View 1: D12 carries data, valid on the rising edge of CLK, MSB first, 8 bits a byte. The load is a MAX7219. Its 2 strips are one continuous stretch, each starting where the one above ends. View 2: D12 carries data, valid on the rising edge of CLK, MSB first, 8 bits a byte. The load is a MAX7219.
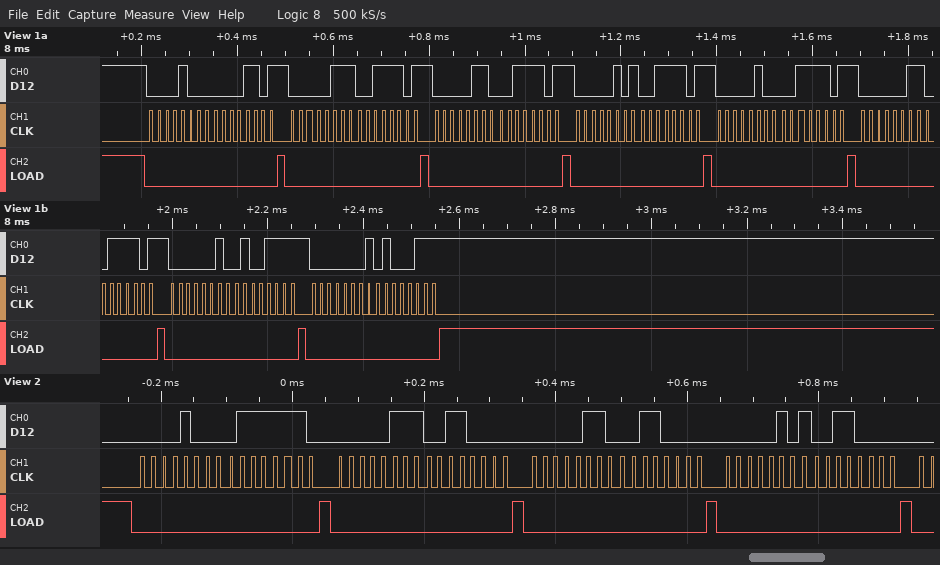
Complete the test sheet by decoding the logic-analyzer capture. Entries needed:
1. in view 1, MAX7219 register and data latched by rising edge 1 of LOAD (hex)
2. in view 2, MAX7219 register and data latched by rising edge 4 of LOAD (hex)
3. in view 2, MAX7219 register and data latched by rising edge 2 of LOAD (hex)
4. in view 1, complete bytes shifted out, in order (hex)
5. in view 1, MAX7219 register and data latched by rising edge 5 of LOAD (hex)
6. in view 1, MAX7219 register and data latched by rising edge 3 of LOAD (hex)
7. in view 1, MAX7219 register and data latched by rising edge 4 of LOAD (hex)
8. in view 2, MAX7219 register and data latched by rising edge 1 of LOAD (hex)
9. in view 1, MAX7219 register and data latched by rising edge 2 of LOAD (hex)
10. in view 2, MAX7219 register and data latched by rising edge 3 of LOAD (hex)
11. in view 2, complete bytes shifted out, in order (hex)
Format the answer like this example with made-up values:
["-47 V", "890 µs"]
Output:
["register 0x8, data 0x0D", "register 0x5, data 0x30", "register 0x7, data 0x30", "0x08 0x0D 0x07 0x3D 0x06 0x3D 0x05 0x3D 0x04 0x3D 0x03 0x3D 0x02 0x4F 0x01 0x47", "register 0x4, data 0x3D", "register 0x6, data 0x3D", "register 0x5, data 0x3D", "register 0x8, data 0x7E", "register 0x7, data 0x3D", "register 0x6, data 0x30", "0x08 0x7E 0x07 0x30 0x06 0x30 0x05 0x30"]
